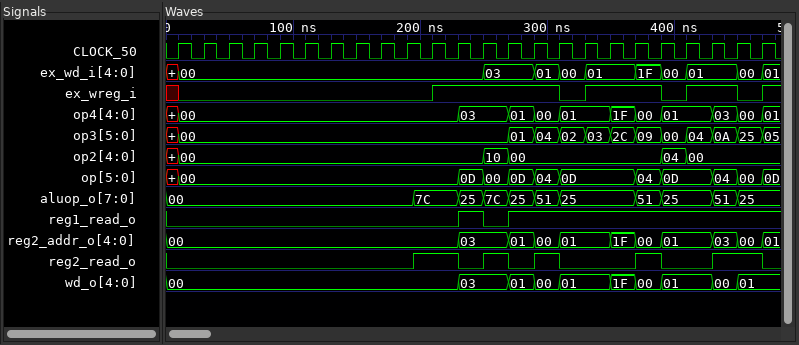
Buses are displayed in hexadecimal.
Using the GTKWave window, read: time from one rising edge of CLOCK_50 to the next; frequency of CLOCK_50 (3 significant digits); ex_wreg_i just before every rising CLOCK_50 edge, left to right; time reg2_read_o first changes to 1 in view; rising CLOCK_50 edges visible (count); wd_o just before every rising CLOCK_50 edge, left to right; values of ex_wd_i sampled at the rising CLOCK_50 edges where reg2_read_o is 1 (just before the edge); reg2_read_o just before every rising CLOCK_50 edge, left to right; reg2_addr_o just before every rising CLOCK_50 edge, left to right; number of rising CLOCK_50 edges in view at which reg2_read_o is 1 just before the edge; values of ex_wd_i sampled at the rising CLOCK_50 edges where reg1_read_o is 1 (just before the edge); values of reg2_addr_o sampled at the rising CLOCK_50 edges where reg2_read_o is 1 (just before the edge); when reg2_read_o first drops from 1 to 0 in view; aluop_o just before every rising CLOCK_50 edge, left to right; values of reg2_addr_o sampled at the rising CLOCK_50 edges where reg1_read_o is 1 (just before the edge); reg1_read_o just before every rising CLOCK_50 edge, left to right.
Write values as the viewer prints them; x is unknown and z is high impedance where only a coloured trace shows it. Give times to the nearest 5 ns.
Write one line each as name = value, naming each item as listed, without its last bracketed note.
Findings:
time from one rising edge of CLOCK_50 to the next = 20 ns
frequency of CLOCK_50 = 50.0 MHz
ex_wreg_i just before every rising CLOCK_50 edge, left to right = x 0 0 0 0 0 0 0 0 0 0 1 1 1 1 1 0 1 1 1 0 1 1 0
time reg2_read_o first changes to 1 in view = 195 ns
rising CLOCK_50 edges visible = 24
wd_o just before every rising CLOCK_50 edge, left to right = 00, 00, 00, 00, 00, 00, 00, 00, 00, 00, 00, 00, 03, 03, 01, 00, 01, 01, 1F, 00, 01, 01, 00, 01
values of ex_wd_i sampled at the rising CLOCK_50 edges where reg2_read_o is 1 = 00, 00, 03, 01, 1F, 01, 00
reg2_read_o just before every rising CLOCK_50 edge, left to right = 0 0 0 0 0 0 0 0 0 0 1 1 0 1 0 1 0 0 0 1 0 0 1 1
reg2_addr_o just before every rising CLOCK_50 edge, left to right = 00, 00, 00, 00, 00, 00, 00, 00, 00, 00, 00, 00, 03, 03, 01, 00, 01, 01, 1F, 00, 01, 01, 03, 00
number of rising CLOCK_50 edges in view at which reg2_read_o is 1 just before the edge = 7
values of ex_wd_i sampled at the rising CLOCK_50 edges where reg1_read_o is 1 = 00, 03, 01, 00, 01, 01, 1F, 00, 01, 01, 00
values of reg2_addr_o sampled at the rising CLOCK_50 edges where reg2_read_o is 1 = 00, 00, 03, 00, 00, 03, 00
when reg2_read_o first drops from 1 to 0 in view = 230 ns
aluop_o just before every rising CLOCK_50 edge, left to right = 00, 00, 00, 00, 00, 00, 00, 00, 00, 00, 7C, 7C, 25, 7C, 25, 51, 25, 25, 25, 51, 25, 25, 51, 25
values of reg2_addr_o sampled at the rising CLOCK_50 edges where reg1_read_o is 1 = 03, 01, 00, 01, 01, 1F, 00, 01, 01, 03, 00
reg1_read_o just before every rising CLOCK_50 edge, left to right = 0 0 0 0 0 0 0 0 0 0 0 0 1 0 1 1 1 1 1 1 1 1 1 1
